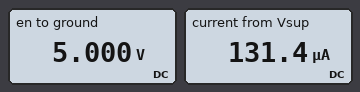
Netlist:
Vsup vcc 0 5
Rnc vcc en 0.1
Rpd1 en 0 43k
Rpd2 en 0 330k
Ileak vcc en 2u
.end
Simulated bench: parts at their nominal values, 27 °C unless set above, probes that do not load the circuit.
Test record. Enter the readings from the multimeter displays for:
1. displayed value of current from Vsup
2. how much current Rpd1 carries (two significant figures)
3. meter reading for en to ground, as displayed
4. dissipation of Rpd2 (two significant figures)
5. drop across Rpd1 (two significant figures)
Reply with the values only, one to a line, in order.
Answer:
131.4 µA
120 µA
5.000 V
76 µW
5.0 V
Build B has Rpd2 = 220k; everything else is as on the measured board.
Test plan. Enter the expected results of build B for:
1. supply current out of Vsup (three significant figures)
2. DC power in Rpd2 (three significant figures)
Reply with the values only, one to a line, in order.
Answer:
139 µA
114 µW
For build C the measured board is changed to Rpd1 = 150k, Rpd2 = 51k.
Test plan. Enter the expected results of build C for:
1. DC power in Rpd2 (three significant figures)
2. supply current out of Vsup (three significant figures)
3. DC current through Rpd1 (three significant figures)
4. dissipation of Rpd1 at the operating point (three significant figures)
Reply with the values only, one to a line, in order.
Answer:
490 µW
131 µA
33.3 µA
167 µW
